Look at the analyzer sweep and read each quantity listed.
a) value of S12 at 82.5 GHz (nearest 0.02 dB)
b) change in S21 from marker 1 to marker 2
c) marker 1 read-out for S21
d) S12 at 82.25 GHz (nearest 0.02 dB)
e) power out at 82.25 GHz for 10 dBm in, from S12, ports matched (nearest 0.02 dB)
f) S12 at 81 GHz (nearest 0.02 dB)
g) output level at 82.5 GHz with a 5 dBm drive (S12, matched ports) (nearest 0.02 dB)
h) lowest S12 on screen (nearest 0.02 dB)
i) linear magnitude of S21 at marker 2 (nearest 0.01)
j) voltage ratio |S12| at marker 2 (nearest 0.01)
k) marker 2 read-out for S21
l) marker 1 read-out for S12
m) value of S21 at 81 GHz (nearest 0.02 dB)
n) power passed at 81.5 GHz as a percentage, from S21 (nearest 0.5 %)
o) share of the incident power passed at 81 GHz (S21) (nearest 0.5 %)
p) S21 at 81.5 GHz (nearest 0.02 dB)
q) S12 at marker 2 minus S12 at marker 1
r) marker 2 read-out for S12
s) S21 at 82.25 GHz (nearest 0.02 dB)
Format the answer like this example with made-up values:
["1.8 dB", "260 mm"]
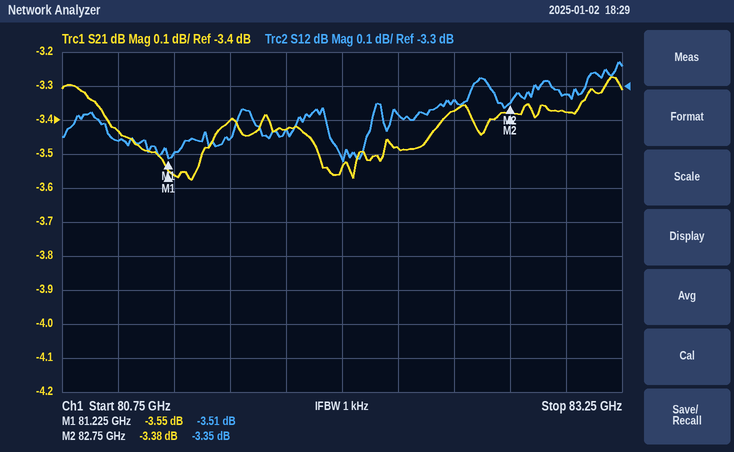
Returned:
["-3.34 dB", "0.17 dB", "-3.55 dB", "-3.38 dB", "6.62 dBm", "-3.46 dB", "1.66 dBm", "-3.52 dB", "0.68", "0.68", "-3.38 dB", "-3.51 dB", "-3.44 dB", "45.5 %", "45.5 %", "-3.40 dB", "0.16 dB", "-3.35 dB", "-3.48 dB"]
